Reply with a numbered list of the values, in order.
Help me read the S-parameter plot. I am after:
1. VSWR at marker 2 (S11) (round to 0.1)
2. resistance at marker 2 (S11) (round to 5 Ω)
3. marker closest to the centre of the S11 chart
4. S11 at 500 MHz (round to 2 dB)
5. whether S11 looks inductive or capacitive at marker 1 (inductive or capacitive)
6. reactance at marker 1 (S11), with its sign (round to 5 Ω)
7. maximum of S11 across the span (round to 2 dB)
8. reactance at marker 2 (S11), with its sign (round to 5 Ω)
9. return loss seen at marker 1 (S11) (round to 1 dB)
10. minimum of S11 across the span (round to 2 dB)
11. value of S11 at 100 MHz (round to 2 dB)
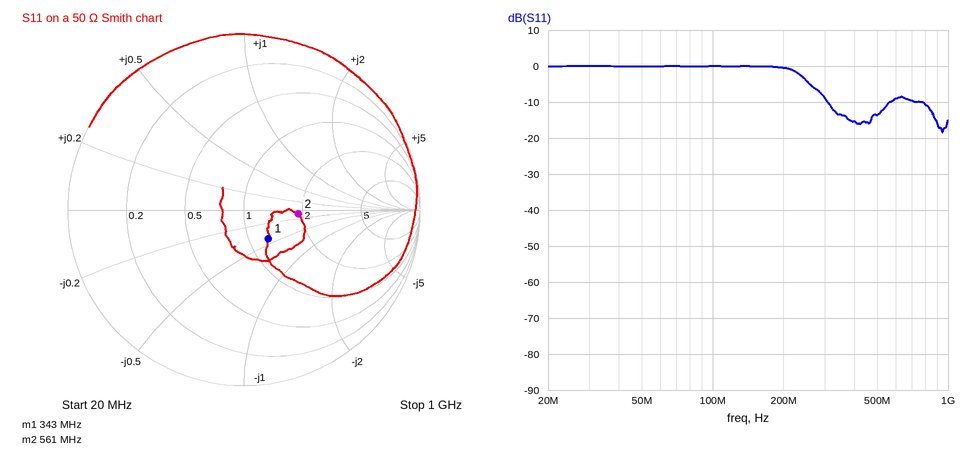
1. 1.9
2. 95 Ω
3. marker 1
4. -14 dB
5. capacitive
6. -20 Ω
7. 0 dB
8. -5 Ω
9. 13 dB
10. -18 dB
11. 0 dB
